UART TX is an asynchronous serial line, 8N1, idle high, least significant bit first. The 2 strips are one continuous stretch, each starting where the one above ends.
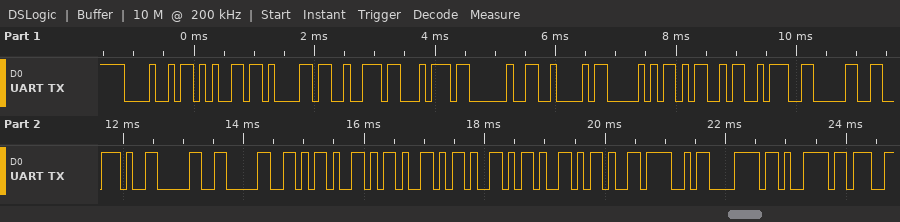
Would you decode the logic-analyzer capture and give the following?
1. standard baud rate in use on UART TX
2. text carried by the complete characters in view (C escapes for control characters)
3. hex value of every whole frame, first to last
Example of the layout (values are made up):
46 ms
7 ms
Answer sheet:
9600 baud
"Heart BPM:0.00-----Oxy"
48 65 61 72 74 20 42 50 4D 3A 30 2E 30 30 2D 2D 2D 2D 2D 4F 78 79
